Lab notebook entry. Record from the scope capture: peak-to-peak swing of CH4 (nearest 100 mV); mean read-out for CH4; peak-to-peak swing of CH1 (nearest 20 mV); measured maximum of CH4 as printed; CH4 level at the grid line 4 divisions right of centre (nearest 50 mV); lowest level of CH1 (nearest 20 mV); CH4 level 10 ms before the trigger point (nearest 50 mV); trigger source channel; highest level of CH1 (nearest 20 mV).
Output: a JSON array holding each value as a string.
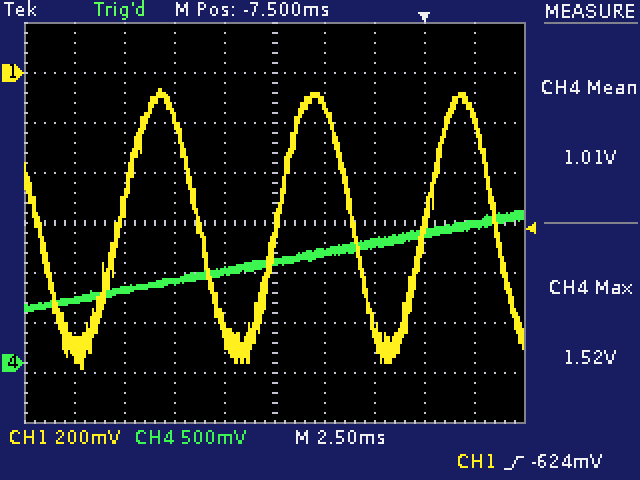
["1.00 V", "1.01 V", "1.12 V", "1.52 V", "1.40 V", "-1.18 V", "900 mV", "CH1", "-60 mV"]
